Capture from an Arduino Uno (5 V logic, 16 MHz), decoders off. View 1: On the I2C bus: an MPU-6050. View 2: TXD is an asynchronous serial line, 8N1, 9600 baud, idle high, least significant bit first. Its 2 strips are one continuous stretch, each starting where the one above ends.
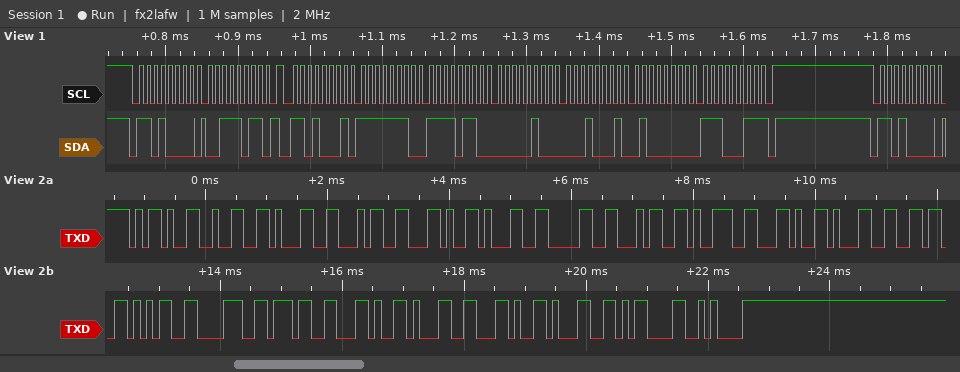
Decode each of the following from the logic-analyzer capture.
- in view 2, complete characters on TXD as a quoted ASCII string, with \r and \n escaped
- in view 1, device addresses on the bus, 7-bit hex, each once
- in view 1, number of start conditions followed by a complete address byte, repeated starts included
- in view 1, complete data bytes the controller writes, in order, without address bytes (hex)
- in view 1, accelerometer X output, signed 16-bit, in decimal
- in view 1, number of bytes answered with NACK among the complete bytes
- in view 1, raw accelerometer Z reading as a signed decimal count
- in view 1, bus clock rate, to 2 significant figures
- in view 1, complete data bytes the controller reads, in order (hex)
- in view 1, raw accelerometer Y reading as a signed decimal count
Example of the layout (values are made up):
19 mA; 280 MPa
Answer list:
"-214,1049,16587,1,1\r\n"; 0x68; 3; 3B; -266; 1; 16611; 100 kHz; FE F6 04 11 40 E3; 1041
